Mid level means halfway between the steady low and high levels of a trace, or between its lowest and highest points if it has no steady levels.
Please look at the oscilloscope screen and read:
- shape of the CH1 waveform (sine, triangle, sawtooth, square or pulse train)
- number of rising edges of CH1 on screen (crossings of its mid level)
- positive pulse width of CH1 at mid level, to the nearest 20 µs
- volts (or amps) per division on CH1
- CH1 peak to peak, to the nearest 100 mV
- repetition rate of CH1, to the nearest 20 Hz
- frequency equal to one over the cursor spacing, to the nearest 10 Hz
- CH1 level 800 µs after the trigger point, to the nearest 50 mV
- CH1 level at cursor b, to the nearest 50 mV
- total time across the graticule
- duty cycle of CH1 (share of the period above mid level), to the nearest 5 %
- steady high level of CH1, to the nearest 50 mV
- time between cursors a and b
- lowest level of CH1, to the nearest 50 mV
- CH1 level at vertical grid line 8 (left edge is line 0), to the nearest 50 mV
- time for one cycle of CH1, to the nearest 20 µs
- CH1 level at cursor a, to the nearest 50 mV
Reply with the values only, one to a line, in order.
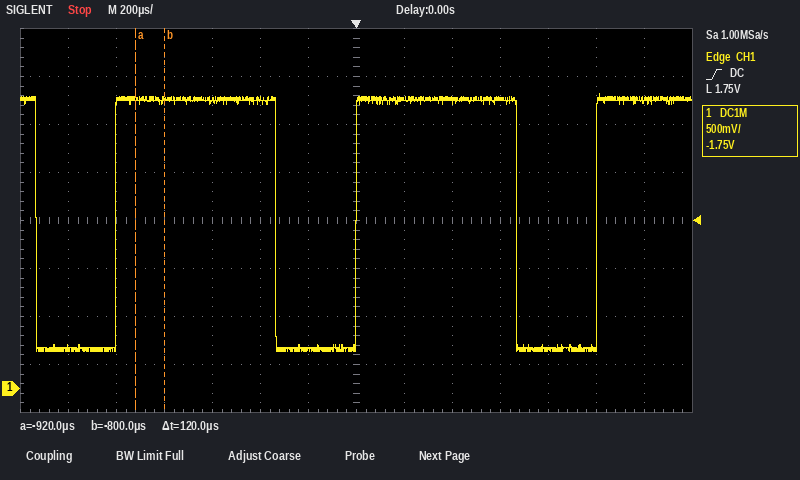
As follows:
pulse train
3
660 µs
500 mV
2.70 V
1.00 kHz
8.33 kHz
400 mV
3.00 V
2.8 ms
65 %
3.00 V
120 µs
400 mV
3.00 V
1.00 ms
3.00 V
